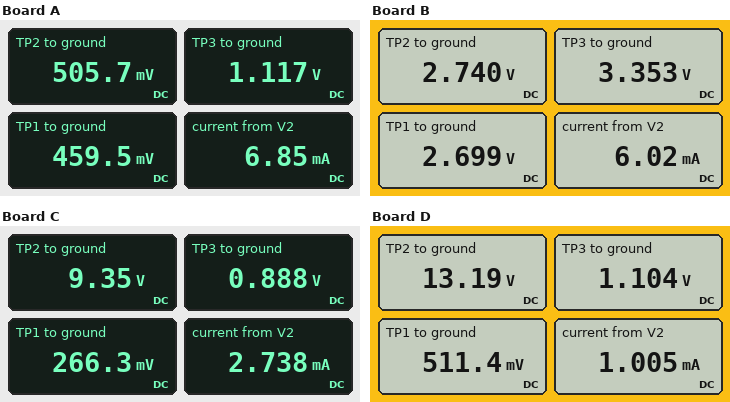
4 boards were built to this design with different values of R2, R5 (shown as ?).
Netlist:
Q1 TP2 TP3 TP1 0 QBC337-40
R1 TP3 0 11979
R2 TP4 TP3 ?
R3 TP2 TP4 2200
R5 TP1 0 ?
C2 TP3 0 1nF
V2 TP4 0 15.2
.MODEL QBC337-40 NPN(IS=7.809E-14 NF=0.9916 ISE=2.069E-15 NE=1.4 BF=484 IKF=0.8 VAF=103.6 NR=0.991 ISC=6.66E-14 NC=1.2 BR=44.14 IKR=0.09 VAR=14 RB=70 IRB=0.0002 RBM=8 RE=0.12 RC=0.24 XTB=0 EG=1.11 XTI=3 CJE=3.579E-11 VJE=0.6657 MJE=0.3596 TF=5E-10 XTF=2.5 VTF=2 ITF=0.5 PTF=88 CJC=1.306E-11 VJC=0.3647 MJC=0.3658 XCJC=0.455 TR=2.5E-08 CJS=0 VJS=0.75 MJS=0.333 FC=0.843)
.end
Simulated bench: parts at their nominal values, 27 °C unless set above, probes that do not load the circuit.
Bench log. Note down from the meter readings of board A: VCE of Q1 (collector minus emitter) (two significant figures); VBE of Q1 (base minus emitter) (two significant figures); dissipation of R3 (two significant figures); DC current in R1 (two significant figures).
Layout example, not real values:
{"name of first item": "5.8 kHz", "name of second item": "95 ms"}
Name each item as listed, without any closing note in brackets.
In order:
{"VCE of Q1 (collector minus emitter)": "46 mV", "VBE of Q1 (base minus emitter)": "660 mV", "dissipation of R3": "98 mW", "DC current in R1": "93 µA"}
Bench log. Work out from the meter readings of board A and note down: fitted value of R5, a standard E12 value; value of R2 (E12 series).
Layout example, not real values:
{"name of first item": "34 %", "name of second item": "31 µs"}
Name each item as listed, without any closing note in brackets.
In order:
{"fitted value of R5, a standard E12 value": "68 Ω", "value of R2": "82 kΩ"}
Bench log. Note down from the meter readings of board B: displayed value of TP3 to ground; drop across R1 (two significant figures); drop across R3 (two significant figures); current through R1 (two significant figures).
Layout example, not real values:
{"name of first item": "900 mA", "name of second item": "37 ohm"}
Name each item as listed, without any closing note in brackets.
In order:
{"displayed value of TP3 to ground": "3.353 V", "drop across R1": "3.4 V", "drop across R3": "12 V", "current through R1": "280 µA"}
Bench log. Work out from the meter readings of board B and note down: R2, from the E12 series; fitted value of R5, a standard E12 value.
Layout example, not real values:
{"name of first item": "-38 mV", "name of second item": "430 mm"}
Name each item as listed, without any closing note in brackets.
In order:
{"R2, from the E12 series": "33 kΩ", "fitted value of R5, a standard E12 value": "470 Ω"}
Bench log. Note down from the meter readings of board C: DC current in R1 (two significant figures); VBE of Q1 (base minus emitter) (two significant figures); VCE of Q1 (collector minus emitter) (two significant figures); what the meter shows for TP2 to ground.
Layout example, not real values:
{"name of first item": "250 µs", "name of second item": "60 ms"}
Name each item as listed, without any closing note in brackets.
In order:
{"DC current in R1": "74 µA", "VBE of Q1 (base minus emitter)": "620 mV", "VCE of Q1 (collector minus emitter)": "9.1 V", "what the meter shows for TP2 to ground": "9.35 V"}
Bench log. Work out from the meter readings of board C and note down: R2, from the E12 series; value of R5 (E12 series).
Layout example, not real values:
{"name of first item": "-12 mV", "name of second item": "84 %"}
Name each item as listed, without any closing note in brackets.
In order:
{"R2, from the E12 series": "180 kΩ", "value of R5": "100 Ω"}
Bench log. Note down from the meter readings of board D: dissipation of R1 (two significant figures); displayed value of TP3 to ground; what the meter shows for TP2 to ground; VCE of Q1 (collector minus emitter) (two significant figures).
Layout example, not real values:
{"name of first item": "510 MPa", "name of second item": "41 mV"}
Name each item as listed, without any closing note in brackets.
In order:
{"dissipation of R1": "100 µW", "displayed value of TP3 to ground": "1.104 V", "what the meter shows for TP2 to ground": "13.19 V", "VCE of Q1 (collector minus emitter)": "13 V"}
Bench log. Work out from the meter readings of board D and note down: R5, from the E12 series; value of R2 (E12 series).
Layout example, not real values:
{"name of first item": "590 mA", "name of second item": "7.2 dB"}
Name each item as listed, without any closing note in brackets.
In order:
{"R5, from the E12 series": "560 Ω", "value of R2": "150 kΩ"}
